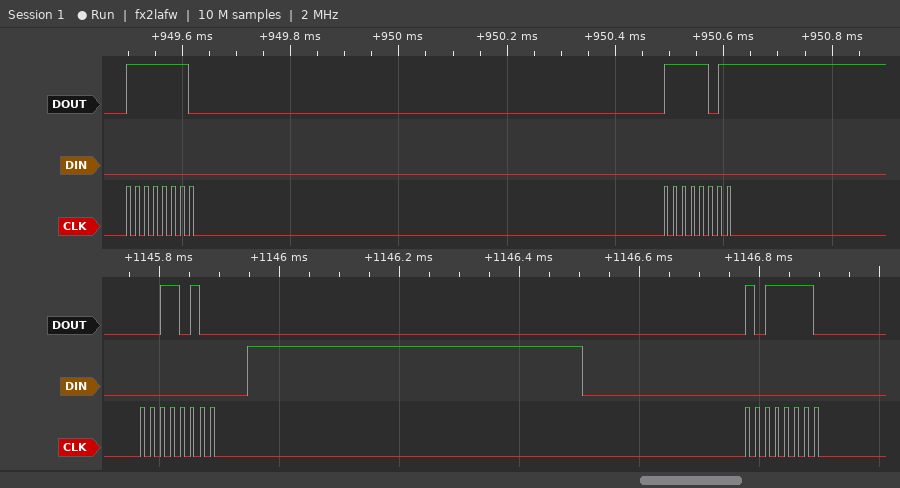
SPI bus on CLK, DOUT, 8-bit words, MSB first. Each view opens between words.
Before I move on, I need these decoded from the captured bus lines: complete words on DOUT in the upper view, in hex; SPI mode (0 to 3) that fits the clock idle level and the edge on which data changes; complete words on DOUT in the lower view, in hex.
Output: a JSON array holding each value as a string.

["FE, FB", "1", "34, BE"]
